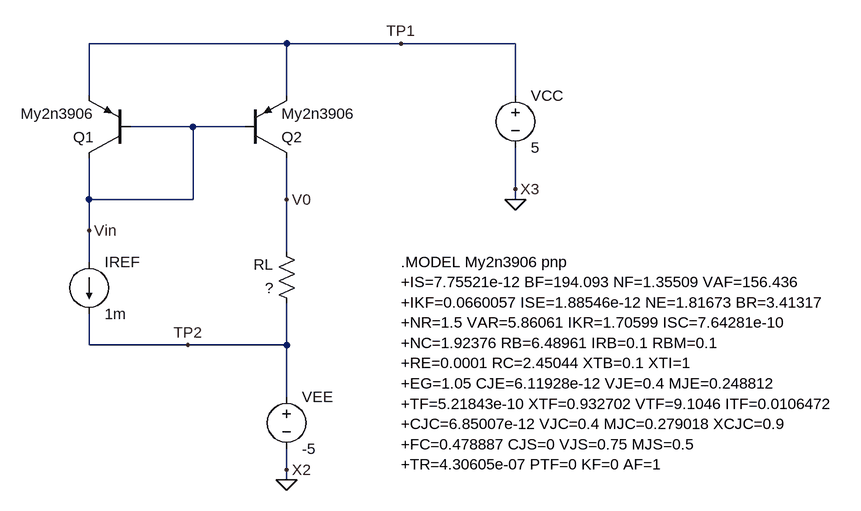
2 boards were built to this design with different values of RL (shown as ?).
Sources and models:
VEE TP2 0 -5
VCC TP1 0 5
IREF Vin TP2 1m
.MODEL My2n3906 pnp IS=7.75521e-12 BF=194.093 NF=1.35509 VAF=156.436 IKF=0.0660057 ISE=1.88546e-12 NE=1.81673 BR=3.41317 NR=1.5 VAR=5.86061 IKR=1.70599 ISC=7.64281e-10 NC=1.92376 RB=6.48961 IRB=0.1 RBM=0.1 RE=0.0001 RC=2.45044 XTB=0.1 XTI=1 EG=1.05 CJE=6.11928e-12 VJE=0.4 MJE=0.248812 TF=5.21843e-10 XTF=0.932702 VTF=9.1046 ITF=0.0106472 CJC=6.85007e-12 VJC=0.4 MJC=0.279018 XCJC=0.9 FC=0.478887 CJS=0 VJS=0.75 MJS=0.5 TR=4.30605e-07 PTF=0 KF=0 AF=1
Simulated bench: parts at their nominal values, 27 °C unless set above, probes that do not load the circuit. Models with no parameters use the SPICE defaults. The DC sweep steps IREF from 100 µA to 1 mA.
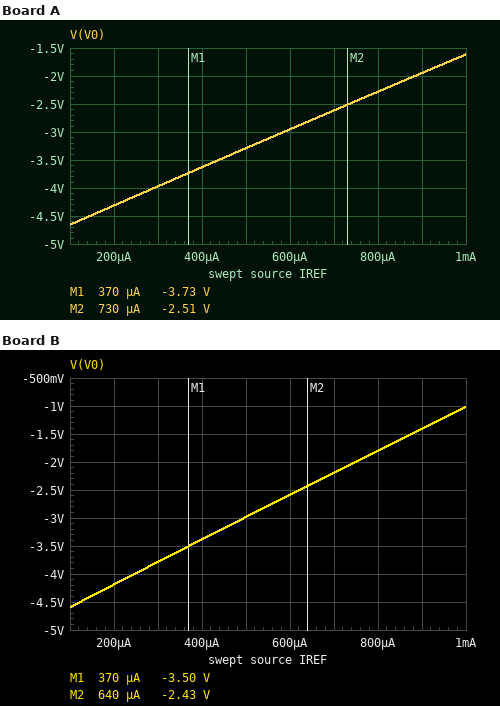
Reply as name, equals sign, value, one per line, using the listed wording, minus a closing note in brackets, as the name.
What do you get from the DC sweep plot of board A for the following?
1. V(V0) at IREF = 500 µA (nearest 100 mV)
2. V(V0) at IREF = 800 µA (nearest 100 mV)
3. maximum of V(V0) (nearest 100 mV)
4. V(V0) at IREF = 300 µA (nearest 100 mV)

V(V0) at IREF = 500 µA = -3.3 V
V(V0) at IREF = 800 µA = -2.3 V
maximum of V(V0) = -1.6 V
V(V0) at IREF = 300 µA = -4.0 V
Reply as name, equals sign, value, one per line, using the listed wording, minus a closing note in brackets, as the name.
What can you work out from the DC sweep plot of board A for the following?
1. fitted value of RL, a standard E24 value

fitted value of RL, a standard E24 value = 3.3 kΩ
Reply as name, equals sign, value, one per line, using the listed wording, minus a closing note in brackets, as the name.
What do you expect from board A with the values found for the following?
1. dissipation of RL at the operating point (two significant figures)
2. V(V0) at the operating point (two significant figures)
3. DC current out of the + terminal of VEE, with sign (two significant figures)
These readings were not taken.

dissipation of RL at the operating point = 3.5 mW
V(V0) at the operating point = -1.6 V
DC current out of the + terminal of VEE, with sign = -2.0 mA
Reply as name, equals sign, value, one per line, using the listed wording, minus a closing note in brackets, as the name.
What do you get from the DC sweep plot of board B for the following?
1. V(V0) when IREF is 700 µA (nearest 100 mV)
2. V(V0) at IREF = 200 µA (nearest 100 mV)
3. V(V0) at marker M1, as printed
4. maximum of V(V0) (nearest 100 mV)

V(V0) when IREF is 700 µA = -2.2 V
V(V0) at IREF = 200 µA = -4.2 V
V(V0) at marker M1, as printed = -3.50 V
maximum of V(V0) = -1.0 V
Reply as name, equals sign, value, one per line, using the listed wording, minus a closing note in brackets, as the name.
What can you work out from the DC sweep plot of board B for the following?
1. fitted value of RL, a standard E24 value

fitted value of RL, a standard E24 value = 3.9 kΩ
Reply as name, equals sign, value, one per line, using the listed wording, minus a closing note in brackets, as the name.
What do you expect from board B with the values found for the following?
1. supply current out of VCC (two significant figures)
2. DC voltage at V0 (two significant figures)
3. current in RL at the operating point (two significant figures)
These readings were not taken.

supply current out of VCC = 2.0 mA
DC voltage at V0 = -1.0 V
current in RL at the operating point = 1.0 mA
